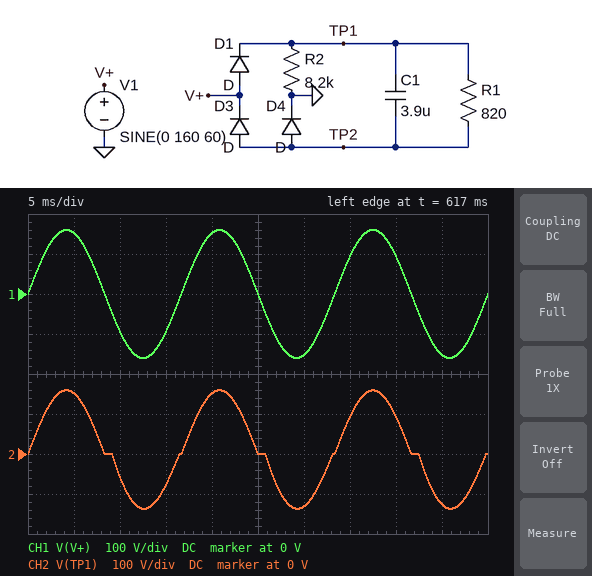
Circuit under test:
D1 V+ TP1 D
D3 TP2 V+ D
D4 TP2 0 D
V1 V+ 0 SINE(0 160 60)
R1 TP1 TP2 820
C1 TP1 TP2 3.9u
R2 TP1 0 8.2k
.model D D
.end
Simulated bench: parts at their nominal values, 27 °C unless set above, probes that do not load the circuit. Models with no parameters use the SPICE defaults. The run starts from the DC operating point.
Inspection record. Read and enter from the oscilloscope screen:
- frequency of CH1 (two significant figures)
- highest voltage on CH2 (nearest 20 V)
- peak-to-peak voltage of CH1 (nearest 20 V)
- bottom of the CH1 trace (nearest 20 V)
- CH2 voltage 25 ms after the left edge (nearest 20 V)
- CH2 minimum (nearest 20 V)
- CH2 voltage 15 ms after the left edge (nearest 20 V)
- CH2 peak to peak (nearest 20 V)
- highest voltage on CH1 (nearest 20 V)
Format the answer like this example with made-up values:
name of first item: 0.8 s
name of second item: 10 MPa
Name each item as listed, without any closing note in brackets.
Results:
frequency of CH1: 60 Hz
highest voltage on CH2: 160 V
peak-to-peak voltage of CH1: 320 V
bottom of the CH1 trace: -160 V
CH2 voltage 25 ms after the left edge: 0 V
CH2 minimum: -140 V
CH2 voltage 15 ms after the left edge: -80 V
CH2 peak to peak: 300 V
highest voltage on CH1: 160 V
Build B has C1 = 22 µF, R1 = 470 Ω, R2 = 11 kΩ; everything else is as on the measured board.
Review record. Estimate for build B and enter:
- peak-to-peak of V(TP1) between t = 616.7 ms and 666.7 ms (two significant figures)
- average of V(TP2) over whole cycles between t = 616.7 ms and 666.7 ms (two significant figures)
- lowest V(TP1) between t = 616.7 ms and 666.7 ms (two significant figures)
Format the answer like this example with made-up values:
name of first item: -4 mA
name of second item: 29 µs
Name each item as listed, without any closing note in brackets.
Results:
peak-to-peak of V(TP1) between t = 616.7 ms and 666.7 ms: 250 V
average of V(TP2) over whole cycles between t = 616.7 ms and 666.7 ms: -67 V
lowest V(TP1) between t = 616.7 ms and 666.7 ms: -87 V
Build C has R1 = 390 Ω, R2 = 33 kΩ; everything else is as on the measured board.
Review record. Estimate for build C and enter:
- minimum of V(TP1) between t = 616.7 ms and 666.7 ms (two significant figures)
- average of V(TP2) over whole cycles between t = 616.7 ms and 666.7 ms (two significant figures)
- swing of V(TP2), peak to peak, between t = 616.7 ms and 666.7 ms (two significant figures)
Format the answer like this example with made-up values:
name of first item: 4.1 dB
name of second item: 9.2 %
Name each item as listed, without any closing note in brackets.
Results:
minimum of V(TP1) between t = 616.7 ms and 666.7 ms: -160 V
average of V(TP2) over whole cycles between t = 616.7 ms and 666.7 ms: -52 V
swing of V(TP2), peak to peak, between t = 616.7 ms and 666.7 ms: 160 V
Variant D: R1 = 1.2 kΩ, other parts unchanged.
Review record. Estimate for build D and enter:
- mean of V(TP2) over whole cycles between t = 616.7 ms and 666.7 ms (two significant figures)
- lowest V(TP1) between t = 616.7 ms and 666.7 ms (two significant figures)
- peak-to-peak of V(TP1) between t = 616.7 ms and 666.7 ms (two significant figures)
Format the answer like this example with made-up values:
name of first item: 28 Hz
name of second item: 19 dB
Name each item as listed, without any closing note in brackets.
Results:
mean of V(TP2) over whole cycles between t = 616.7 ms and 666.7 ms: -58 V
lowest V(TP1) between t = 616.7 ms and 666.7 ms: -120 V
peak-to-peak of V(TP1) between t = 616.7 ms and 666.7 ms: 280 V
